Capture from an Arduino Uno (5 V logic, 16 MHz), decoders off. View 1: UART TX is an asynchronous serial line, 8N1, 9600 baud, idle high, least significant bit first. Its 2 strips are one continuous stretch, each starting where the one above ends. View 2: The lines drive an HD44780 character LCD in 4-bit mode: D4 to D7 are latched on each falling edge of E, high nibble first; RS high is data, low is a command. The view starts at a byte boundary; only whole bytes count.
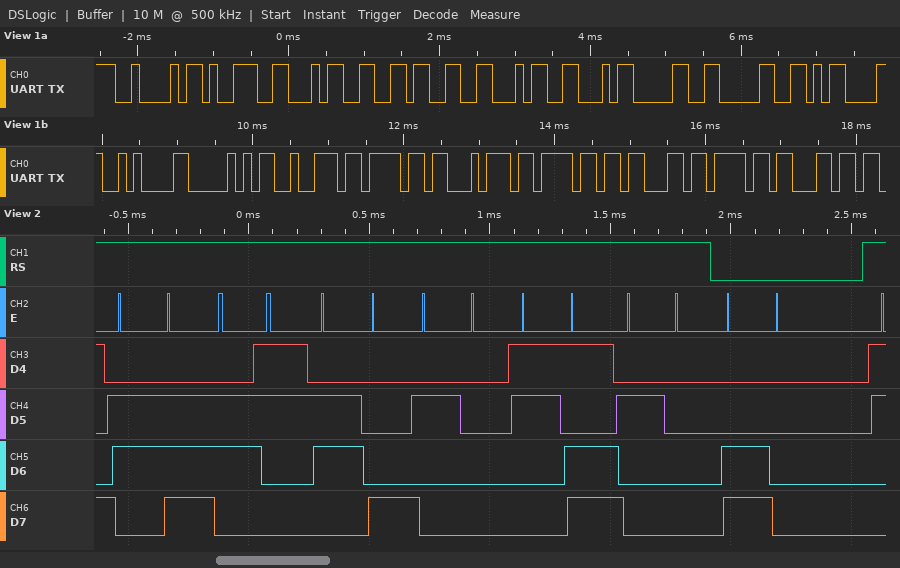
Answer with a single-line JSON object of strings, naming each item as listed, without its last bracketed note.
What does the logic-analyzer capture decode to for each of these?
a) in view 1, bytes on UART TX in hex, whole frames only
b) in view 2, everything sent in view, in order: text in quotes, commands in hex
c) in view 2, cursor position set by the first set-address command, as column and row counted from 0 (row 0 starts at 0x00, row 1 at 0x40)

{"in view 1, bytes on UART TX in hex, whole frames only": "42 39 34 36 46 46 30 30 0D 0A 50 72 6F 74 6F 63 6F 6C", "in view 2, everything sent in view, in order: text in quotes, commands in hex": "\"nch = \" 0xC0", "in view 2, cursor position set by the first set-address command, as column and row counted from 0": "column 0, row 1"}
